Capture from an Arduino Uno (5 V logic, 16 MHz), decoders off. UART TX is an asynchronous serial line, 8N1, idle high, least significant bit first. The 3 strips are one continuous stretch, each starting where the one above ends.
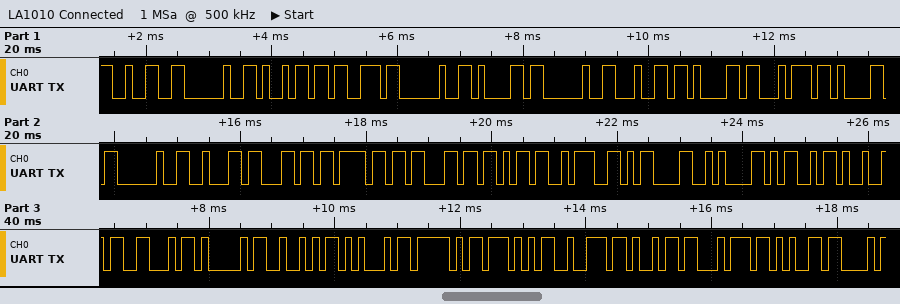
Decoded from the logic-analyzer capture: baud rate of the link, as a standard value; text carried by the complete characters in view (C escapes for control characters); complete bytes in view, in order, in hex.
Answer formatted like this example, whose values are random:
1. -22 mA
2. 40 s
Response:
1. 9600 baud
2. "2 is a data block:\r\nMIFARE_Write"
3. 0x32 0x20 0x69 0x73 0x20 0x61 0x20 0x64 0x61 0x74 0x61 0x20 0x62 0x6C 0x6F 0x63 0x6B 0x3A 0x0D 0x0A 0x4D 0x49 0x46 0x41 0x52 0x45 0x5F 0x57 0x72 0x69 0x74 0x65
